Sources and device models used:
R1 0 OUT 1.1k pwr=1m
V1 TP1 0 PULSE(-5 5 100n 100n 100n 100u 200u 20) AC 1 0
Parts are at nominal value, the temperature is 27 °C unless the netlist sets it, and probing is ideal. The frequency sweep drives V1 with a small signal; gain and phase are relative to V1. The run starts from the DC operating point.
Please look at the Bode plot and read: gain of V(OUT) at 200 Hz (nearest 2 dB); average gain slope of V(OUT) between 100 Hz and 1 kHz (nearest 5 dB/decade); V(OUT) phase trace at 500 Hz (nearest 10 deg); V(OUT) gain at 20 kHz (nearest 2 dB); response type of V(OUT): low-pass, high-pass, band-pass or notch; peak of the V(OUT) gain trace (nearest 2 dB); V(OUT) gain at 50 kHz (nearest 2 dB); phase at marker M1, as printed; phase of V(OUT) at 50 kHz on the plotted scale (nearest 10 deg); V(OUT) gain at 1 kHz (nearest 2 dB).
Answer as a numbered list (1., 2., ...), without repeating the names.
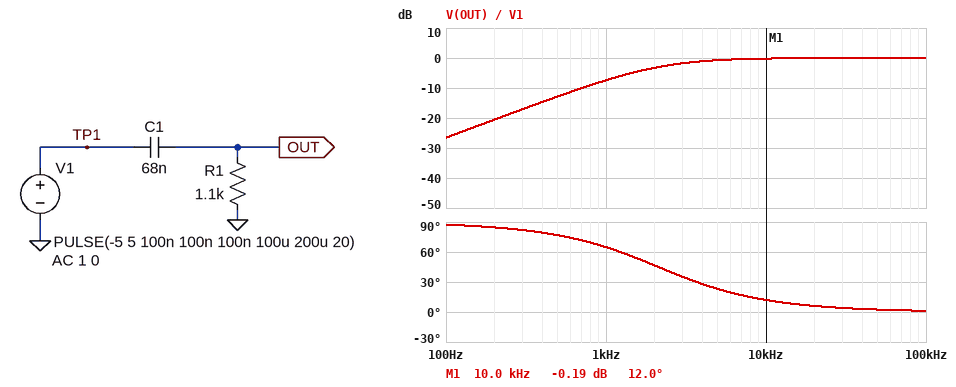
1. -20 dB
2. 20 dB/decade
3. 80 deg
4. 0 dB
5. high-pass
6. 0 dB
7. 0 dB
8. 12.0 deg
9. 0 deg
10. -8 dB
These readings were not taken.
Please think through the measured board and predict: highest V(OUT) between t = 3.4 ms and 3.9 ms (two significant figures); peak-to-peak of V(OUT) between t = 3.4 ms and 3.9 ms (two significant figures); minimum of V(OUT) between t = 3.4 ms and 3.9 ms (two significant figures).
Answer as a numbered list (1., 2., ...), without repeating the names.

1. 7.9 V
2. 16 V
3. -7.9 V
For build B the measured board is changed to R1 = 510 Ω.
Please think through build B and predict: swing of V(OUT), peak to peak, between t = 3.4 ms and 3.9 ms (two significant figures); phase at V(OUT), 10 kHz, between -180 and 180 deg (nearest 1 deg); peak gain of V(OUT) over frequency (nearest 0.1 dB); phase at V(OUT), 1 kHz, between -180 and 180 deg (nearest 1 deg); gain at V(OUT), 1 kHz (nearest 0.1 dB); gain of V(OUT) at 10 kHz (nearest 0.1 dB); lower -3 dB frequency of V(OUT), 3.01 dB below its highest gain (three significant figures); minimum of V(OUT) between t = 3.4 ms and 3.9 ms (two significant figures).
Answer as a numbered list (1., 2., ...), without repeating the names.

1. 19 V
2. 25 deg
3. 0 dB
4. 78 deg
5. -13.4 dB
6. -0.8 dB
7. 4.59 kHz
8. -9.5 V
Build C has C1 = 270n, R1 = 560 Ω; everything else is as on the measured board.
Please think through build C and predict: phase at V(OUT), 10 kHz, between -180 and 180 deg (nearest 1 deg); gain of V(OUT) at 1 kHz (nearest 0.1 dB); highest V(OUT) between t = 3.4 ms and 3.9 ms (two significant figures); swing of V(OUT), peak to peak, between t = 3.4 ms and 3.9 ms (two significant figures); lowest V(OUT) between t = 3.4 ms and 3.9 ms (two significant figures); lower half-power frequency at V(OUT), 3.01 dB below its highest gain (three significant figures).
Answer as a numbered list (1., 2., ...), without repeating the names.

1. 6 deg
2. -3.2 dB
3. 6.6 V
4. 13 V
5. -6.6 V
6. 1.05 kHz
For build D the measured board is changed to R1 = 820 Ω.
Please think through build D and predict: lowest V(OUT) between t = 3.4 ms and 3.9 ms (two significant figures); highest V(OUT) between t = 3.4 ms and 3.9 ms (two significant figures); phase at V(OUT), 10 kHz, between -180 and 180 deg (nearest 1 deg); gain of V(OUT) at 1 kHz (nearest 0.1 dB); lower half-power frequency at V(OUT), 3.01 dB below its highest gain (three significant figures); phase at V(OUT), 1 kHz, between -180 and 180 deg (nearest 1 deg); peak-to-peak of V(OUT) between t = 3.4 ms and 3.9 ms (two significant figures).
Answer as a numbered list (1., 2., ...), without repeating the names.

1. -8.6 V
2. 8.6 V
3. 16 deg
4. -9.6 dB
5. 2.85 kHz
6. 71 deg
7. 17 V
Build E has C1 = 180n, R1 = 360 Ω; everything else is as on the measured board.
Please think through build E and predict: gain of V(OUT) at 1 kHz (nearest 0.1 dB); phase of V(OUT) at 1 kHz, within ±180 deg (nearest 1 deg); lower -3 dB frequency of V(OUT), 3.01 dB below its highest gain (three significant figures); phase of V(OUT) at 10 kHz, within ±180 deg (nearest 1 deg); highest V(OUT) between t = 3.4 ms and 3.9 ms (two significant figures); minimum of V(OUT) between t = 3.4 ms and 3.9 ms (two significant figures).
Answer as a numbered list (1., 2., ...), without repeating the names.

1. -8.5 dB
2. 68 deg
3. 2.46 kHz
4. 14 deg
5. 8.2 V
6. -8.2 V
